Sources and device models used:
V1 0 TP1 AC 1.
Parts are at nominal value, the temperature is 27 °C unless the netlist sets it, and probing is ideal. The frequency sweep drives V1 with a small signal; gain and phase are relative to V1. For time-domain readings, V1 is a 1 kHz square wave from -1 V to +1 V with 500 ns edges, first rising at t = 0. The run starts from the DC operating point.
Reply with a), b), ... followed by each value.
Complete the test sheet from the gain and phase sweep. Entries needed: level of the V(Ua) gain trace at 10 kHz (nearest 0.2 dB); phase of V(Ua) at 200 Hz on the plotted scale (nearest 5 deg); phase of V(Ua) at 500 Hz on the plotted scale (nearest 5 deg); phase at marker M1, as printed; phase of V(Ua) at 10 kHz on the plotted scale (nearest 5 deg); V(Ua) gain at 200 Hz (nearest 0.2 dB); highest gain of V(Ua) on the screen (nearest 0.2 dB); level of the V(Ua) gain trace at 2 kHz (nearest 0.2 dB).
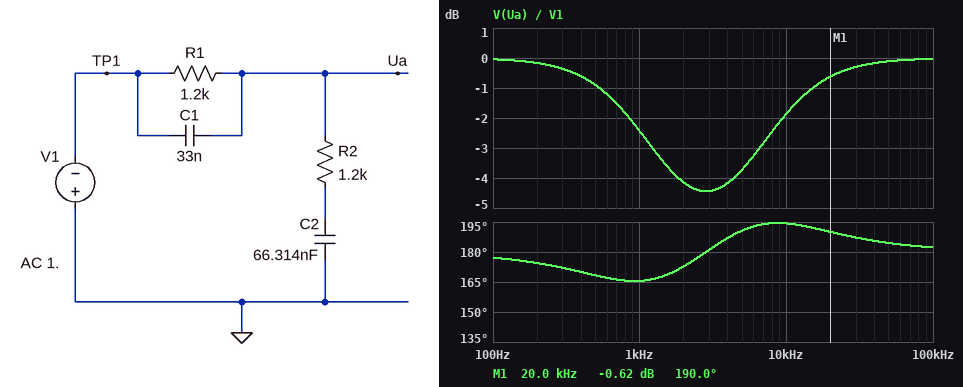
a) -1.8 dB
b) 175 deg
c) 170 deg
d) 190.0 deg
e) 195 deg
f) -0.2 dB
g) 0 dB
h) -4.2 dB
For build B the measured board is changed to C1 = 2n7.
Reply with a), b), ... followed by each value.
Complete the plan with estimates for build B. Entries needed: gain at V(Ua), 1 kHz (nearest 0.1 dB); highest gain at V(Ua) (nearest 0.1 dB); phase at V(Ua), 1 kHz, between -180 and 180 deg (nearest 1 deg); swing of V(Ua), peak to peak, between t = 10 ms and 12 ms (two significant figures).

a) -2.1 dB
b) 0 dB
c) 162 deg
d) 1.9 V
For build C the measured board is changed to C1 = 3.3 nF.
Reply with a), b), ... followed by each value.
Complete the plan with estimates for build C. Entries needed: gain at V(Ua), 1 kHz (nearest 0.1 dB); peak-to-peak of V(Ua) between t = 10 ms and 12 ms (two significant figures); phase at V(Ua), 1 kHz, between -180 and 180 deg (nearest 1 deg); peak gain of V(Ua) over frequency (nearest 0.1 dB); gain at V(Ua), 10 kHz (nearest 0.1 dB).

a) -2.1 dB
b) 1.9 V
c) 162 deg
d) 0 dB
e) -5.8 dB
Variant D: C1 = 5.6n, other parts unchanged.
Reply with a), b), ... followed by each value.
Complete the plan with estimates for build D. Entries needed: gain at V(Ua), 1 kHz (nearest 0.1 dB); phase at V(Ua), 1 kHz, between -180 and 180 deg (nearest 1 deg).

a) -2.1 dB
b) 162 deg
